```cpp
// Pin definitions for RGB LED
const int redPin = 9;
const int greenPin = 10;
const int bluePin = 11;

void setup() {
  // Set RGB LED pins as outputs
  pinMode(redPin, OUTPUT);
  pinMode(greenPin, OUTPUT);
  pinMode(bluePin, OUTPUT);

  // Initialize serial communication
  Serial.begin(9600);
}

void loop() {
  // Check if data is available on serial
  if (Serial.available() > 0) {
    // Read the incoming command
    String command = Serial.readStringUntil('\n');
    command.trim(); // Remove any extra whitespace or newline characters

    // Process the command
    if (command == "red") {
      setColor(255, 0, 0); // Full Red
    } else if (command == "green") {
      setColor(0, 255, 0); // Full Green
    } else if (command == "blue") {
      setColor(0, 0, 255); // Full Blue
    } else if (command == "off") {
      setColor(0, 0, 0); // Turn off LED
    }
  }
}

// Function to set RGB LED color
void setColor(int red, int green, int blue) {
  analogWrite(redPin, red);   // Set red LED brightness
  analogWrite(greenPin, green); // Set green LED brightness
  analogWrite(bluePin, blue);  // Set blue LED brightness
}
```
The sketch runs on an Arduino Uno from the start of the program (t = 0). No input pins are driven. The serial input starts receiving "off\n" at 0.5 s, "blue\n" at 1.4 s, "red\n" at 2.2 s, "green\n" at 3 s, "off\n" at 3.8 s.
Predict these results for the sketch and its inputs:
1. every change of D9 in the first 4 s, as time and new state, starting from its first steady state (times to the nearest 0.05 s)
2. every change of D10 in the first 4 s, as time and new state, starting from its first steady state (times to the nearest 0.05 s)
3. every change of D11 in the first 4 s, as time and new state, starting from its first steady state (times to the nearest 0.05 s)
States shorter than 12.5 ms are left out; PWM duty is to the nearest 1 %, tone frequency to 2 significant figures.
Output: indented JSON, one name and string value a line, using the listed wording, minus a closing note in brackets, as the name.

{
  "every change of D9 in the first 4 s, as time and new state, starting from its first steady state": "0 s low; 2.2 s high; 3 s low",
  "every change of D10 in the first 4 s, as time and new state, starting from its first steady state": "0 s low; 3 s high; 3.8 s low",
  "every change of D11 in the first 4 s, as time and new state, starting from its first steady state": "0 s low; 1.4 s high; 2.2 s low"
}
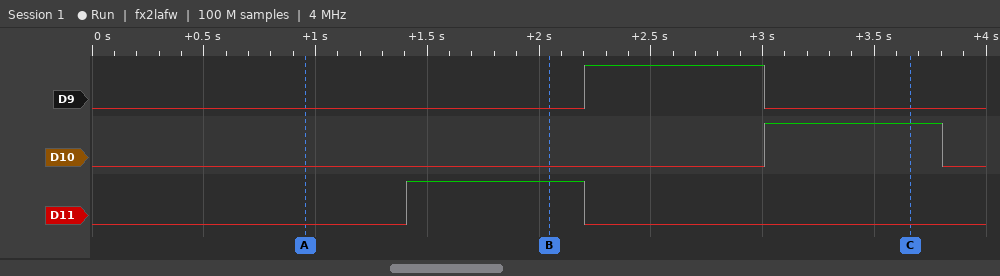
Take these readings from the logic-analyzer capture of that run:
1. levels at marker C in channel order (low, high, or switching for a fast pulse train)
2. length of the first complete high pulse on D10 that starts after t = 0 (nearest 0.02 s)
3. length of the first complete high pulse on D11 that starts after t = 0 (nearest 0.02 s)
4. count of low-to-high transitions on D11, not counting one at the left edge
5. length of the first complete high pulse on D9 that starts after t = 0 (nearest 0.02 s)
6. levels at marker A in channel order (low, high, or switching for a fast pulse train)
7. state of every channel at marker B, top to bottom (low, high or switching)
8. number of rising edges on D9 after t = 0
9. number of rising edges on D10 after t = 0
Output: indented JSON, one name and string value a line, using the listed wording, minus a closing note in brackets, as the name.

{
  "levels at marker C in channel order": "D9 low, D10 high, D11 low",
  "length of the first complete high pulse on D10 that starts after t = 0": "0.80 s",
  "length of the first complete high pulse on D11 that starts after t = 0": "0.80 s",
  "count of low-to-high transitions on D11, not counting one at the left edge": "1",
  "length of the first complete high pulse on D9 that starts after t = 0": "0.80 s",
  "levels at marker A in channel order": "D9 low, D10 low, D11 low",
  "state of every channel at marker B, top to bottom": "D9 low, D10 low, D11 high",
  "number of rising edges on D9 after t = 0": "1",
  "number of rising edges on D10 after t = 0": "1"
}
